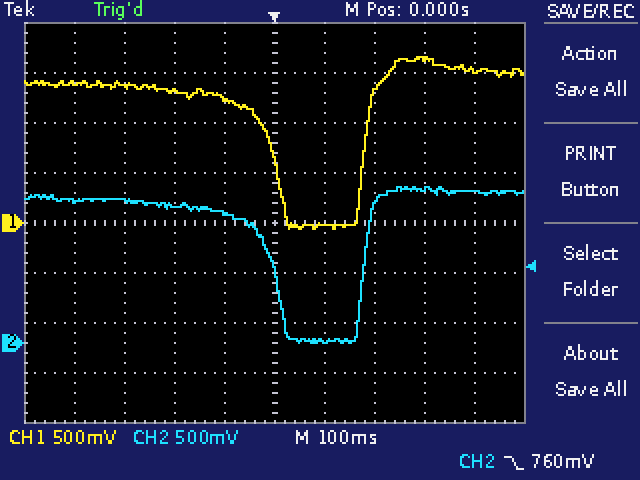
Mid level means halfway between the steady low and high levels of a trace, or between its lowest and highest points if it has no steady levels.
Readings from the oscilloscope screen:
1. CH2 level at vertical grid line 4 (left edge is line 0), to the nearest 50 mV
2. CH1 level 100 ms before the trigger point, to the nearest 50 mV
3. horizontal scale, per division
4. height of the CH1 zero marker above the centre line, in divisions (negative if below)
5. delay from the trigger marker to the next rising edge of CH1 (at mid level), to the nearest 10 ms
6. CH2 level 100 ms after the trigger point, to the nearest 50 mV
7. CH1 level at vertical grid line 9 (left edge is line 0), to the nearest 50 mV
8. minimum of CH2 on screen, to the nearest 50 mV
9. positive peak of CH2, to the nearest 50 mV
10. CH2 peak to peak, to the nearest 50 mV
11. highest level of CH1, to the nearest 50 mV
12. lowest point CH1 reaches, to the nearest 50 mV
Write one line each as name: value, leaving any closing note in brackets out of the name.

CH2 level at vertical grid line 4 (left edge is line 0), to the nearest 50 mV: 1.30 V
CH1 level 100 ms before the trigger point, to the nearest 50 mV: 1.25 V
horizontal scale, per division: 100 ms
height of the CH1 zero marker above the centre line, in divisions: 0.0 div
delay from the trigger marker to the next rising edge of CH1 (at mid level), to the nearest 10 ms: 180 ms
CH2 level 100 ms after the trigger point, to the nearest 50 mV: 0 mV
CH1 level at vertical grid line 9 (left edge is line 0), to the nearest 50 mV: 1.55 V
minimum of CH2 on screen, to the nearest 50 mV: 0 mV
positive peak of CH2, to the nearest 50 mV: 1.55 V
CH2 peak to peak, to the nearest 50 mV: 1.55 V
highest level of CH1, to the nearest 50 mV: 1.65 V
lowest point CH1 reaches, to the nearest 50 mV: -50 mV
